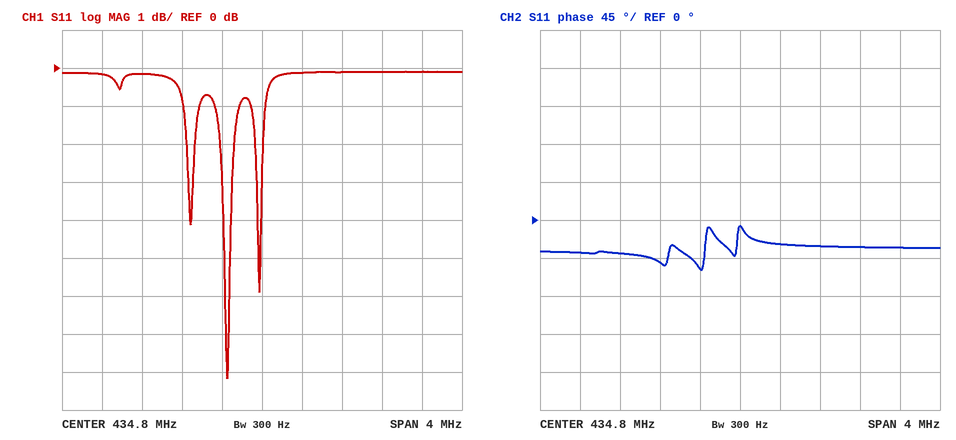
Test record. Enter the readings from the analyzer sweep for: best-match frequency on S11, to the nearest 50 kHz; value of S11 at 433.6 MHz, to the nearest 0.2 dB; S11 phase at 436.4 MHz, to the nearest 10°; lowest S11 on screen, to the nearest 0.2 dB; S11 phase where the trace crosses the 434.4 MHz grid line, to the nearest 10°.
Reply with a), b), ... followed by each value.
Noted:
a) 434.45 MHz
b) -0.2 dB
c) -30°
d) -8.2 dB
e) -60°
